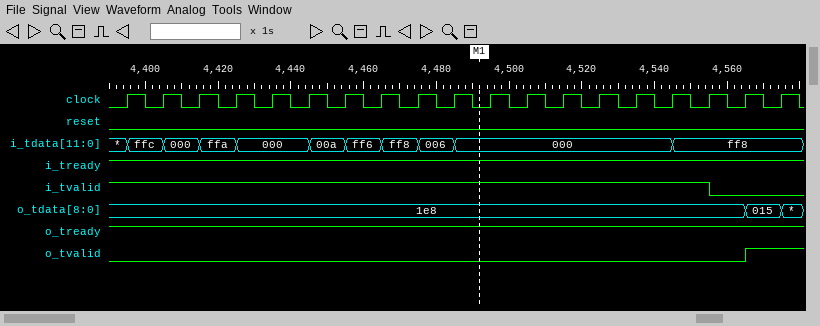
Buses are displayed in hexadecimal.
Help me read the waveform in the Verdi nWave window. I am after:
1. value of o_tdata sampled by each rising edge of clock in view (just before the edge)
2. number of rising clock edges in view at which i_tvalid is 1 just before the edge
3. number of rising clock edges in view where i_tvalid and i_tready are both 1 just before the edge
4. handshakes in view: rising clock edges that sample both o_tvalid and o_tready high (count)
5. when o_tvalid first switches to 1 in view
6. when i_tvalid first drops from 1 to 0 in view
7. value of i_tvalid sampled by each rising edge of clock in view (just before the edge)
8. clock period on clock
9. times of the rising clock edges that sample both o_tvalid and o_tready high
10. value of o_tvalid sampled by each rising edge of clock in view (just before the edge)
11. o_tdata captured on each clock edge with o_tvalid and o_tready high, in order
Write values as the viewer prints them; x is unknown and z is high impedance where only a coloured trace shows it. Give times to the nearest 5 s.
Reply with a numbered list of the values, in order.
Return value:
1. 1e8, 1e8, 1e8, 1e8, 1e8, 1e8, 1e8, 1e8, 1e8, 1e8, 1e8, 1e8, 1e8, 1e8, 1e8, 1e8, 1e8, 1e8, 015
2. 17
3. 17
4. 1
5. 4565 s
6. 4555 s
7. 1 1 1 1 1 1 1 1 1 1 1 1 1 1 1 1 1 0 0
8. 10 s
9. 4575 s
10. 0 0 0 0 0 0 0 0 0 0 0 0 0 0 0 0 0 0 1
11. 015
